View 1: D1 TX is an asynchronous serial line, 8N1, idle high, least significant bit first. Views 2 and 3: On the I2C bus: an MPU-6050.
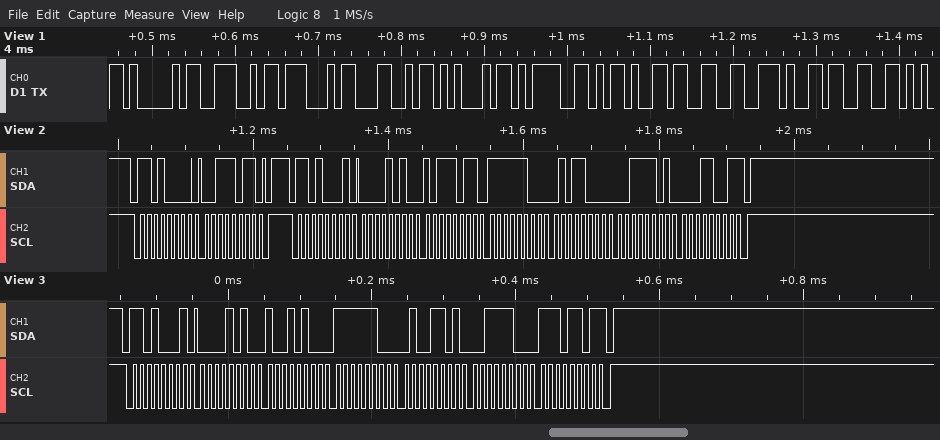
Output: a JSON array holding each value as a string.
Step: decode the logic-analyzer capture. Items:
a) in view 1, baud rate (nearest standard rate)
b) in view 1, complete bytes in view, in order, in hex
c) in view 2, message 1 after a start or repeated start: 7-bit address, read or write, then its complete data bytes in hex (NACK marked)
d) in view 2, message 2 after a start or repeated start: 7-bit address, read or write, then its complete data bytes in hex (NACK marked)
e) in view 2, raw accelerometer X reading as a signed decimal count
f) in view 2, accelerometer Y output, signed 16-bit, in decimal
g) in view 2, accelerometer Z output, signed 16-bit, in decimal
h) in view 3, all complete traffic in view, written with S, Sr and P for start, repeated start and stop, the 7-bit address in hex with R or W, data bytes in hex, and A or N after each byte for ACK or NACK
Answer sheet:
["115200 baud", "0x41 0x4E 0x47 0x4C 0x45 0x3D 0x2D 0x33 0x2E 0x33", "0x68 write: 3B", "0x68 read: 0A BB FC 58 3D 19 NACK", "2747", "-936", "15641", "S 68R A 0A A 94 A FC A 4D A 3C A ED N P"]
